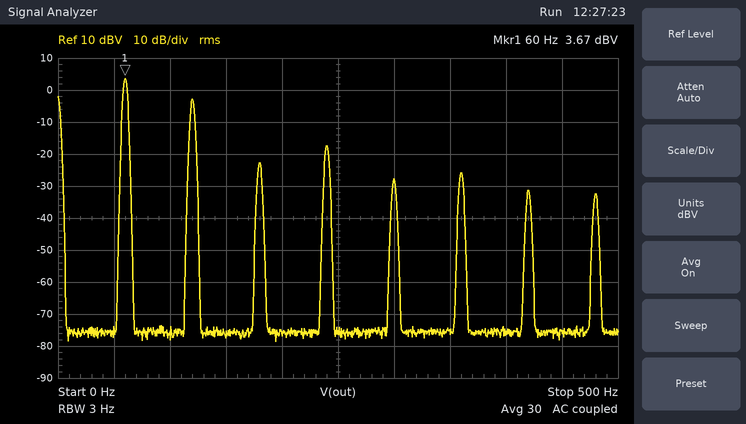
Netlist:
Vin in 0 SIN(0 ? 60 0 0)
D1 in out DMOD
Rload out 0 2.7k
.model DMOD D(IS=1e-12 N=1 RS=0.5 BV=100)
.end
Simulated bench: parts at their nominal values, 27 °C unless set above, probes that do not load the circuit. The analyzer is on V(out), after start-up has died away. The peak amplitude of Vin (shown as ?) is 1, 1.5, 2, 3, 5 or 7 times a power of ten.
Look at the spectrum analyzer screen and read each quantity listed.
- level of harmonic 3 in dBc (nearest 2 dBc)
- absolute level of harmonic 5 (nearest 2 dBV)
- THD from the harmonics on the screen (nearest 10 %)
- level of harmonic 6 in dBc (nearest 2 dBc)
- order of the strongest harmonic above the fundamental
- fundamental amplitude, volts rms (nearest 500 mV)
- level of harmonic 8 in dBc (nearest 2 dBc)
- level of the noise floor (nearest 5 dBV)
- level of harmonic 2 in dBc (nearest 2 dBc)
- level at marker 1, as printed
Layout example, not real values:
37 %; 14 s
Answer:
-26 dBc; -28 dBV; 50 %; -30 dBc; 2; 1.5 V; -36 dBc; -75 dBV; -6 dBc; 3.67 dBV
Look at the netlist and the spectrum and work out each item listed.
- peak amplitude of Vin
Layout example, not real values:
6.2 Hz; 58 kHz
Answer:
5 V
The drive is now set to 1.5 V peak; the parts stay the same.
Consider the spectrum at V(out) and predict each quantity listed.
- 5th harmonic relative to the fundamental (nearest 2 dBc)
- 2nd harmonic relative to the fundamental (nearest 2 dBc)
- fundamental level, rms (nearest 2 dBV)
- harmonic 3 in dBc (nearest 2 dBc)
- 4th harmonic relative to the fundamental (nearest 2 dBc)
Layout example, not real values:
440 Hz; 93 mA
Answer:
-22 dBc; -4 dBc; -10 dBV; -14 dBc; -26 dBc
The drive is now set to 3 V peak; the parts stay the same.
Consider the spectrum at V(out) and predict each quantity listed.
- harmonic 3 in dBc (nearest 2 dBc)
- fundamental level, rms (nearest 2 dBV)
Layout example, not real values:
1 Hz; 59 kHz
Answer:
-22 dBc; -2 dBV
